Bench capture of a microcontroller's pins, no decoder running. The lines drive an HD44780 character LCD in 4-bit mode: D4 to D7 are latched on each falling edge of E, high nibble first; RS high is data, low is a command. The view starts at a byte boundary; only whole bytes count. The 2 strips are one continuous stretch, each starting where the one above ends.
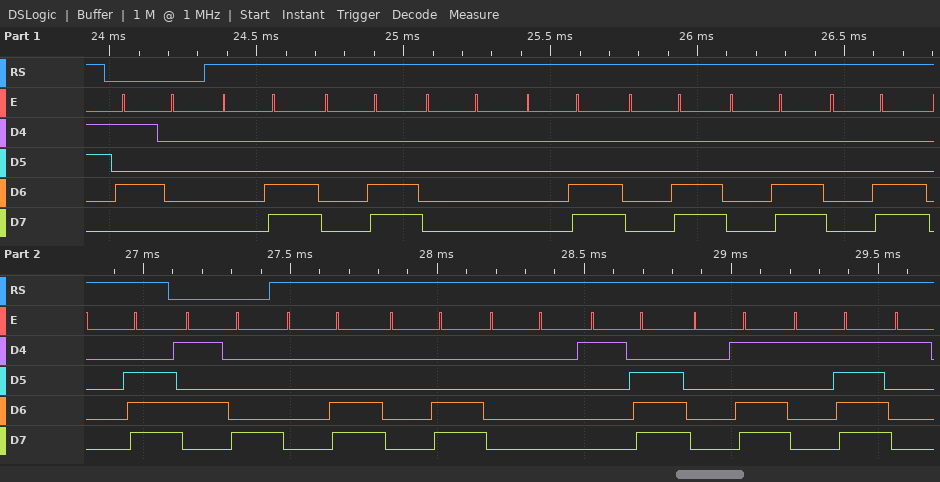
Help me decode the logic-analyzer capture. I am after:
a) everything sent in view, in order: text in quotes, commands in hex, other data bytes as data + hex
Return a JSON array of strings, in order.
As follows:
["0x50 data 0C 0C 00 0C 0C 0C 0C 0E 0x58 data 0C 0C 00 1E 0D 1F"]
